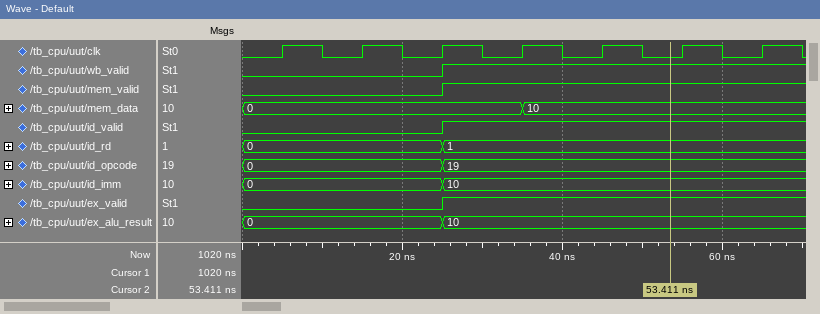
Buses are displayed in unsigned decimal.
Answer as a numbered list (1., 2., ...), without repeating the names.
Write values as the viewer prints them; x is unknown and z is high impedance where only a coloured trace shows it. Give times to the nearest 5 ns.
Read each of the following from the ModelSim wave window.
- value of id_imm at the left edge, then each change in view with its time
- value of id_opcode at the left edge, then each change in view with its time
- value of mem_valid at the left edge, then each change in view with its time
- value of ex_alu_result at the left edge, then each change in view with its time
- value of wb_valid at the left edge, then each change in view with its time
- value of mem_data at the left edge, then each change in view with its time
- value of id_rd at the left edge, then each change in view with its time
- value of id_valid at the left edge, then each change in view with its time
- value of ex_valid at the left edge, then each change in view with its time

1. 0, 10 at 25 ns
2. 0, 19 at 25 ns
3. 0, 1 at 25 ns
4. 0, 10 at 25 ns
5. 0, 1 at 25 ns
6. 0, 10 at 35 ns
7. 0, 1 at 25 ns
8. 0, 1 at 25 ns
9. 0, 1 at 25 ns
